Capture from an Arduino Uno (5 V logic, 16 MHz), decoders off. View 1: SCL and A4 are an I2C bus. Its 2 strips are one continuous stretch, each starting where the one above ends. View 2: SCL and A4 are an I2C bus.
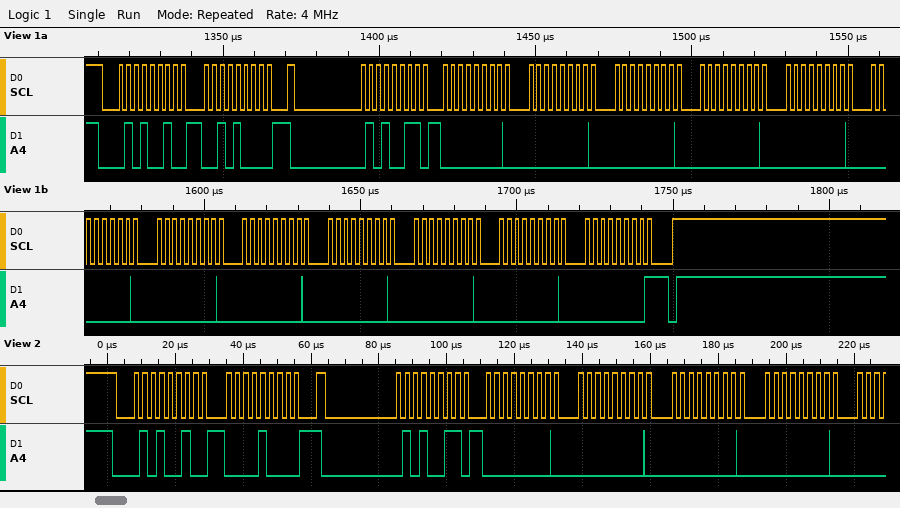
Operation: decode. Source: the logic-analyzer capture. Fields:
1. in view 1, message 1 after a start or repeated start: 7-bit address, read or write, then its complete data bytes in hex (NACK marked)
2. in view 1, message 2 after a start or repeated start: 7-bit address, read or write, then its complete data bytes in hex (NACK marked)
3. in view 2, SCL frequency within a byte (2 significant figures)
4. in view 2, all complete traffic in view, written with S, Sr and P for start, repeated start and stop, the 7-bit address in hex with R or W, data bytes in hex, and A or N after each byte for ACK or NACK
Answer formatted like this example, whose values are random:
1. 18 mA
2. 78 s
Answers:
1. 0x29 write: 28
2. 0x29 read: 00 00 00 00 00 00 00 00 00 00 00 00 NACK
3. 400 kHz
4. S 29W A 08 A Sr 29R A 00 A 00 A 00 A 00 A
